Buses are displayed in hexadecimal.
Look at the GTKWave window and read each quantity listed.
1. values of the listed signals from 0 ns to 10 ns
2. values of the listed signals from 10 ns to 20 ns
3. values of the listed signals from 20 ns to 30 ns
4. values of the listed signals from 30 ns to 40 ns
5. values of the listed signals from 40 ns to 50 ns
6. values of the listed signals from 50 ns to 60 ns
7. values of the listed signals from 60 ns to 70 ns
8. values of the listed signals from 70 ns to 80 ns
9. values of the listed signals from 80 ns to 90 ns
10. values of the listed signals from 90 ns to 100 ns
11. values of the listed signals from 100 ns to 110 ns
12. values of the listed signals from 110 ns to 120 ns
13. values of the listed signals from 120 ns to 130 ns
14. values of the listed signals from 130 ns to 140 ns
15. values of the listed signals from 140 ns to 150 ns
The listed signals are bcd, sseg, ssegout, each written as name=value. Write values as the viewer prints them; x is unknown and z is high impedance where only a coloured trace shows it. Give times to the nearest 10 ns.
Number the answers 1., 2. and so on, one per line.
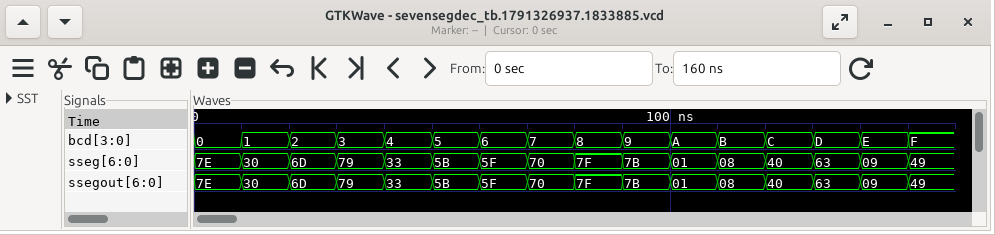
1. bcd=0, sseg=7E, ssegout=7E
2. bcd=1, sseg=30, ssegout=30
3. bcd=2, sseg=6D, ssegout=6D
4. bcd=3, sseg=79, ssegout=79
5. bcd=4, sseg=33, ssegout=33
6. bcd=5, sseg=5B, ssegout=5B
7. bcd=6, sseg=5F, ssegout=5F
8. bcd=7, sseg=70, ssegout=70
9. bcd=8, sseg=7F, ssegout=7F
10. bcd=9, sseg=7B, ssegout=7B
11. bcd=A, sseg=01, ssegout=01
12. bcd=B, sseg=08, ssegout=08
13. bcd=C, sseg=40, ssegout=40
14. bcd=D, sseg=63, ssegout=63
15. bcd=E, sseg=09, ssegout=09
